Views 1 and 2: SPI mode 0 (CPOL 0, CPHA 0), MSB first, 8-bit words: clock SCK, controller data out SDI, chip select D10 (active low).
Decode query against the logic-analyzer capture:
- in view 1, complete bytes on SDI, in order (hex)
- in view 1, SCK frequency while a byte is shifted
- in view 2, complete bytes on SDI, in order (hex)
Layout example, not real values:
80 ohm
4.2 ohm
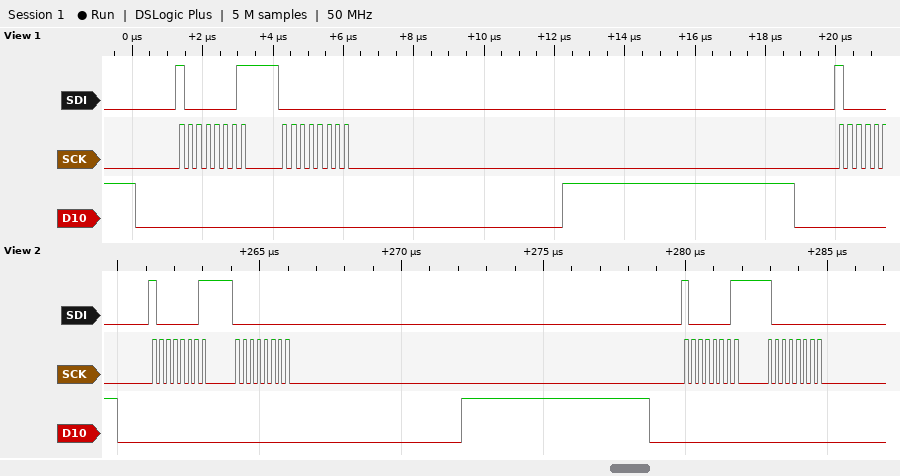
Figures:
81 00
4 MHz
81 00 81 80
